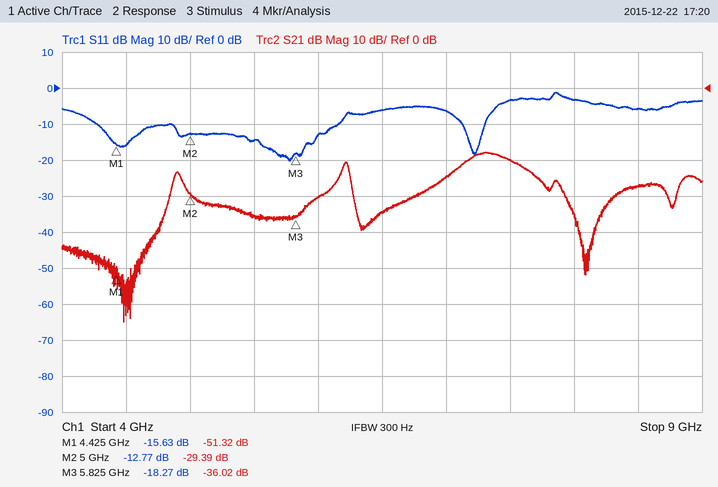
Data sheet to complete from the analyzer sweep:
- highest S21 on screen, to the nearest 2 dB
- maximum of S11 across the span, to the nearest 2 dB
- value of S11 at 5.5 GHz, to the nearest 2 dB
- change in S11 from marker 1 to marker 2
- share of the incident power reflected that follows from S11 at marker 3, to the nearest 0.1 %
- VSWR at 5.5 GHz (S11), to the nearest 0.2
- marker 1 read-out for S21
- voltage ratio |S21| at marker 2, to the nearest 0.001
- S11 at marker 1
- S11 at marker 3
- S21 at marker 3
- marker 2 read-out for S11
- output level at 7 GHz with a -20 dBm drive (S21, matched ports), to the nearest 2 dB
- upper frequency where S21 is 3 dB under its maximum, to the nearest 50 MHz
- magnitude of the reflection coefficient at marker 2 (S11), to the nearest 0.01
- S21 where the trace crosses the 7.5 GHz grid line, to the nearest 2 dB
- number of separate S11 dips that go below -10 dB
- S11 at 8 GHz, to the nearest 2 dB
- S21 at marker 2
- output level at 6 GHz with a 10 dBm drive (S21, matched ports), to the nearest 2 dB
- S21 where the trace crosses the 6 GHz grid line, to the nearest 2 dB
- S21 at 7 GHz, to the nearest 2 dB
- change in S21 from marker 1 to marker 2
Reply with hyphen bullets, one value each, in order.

- -18 dB
- -2 dB
- -14 dB
- 2.86 dB
- 1.5 %
- 1.4
- -51.32 dB
- 0.034
- -15.63 dB
- -18.27 dB
- -36.02 dB
- -12.77 dB
- -44 dBm
- 7.55 GHz
- 0.23
- -20 dB
- 3
- -4 dB
- -29.39 dB
- -20 dBm
- -30 dB
- -24 dB
- 21.93 dB
